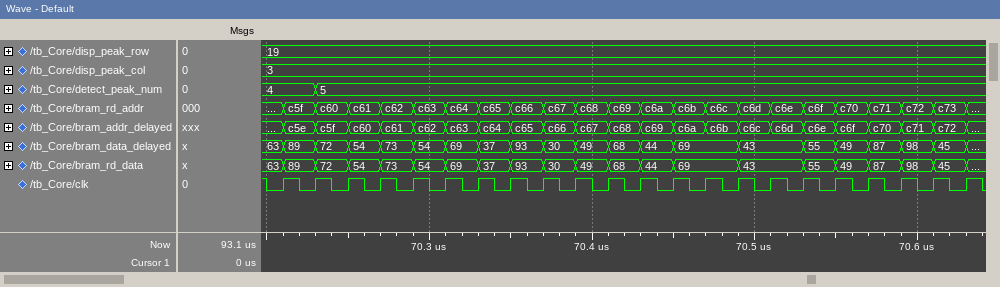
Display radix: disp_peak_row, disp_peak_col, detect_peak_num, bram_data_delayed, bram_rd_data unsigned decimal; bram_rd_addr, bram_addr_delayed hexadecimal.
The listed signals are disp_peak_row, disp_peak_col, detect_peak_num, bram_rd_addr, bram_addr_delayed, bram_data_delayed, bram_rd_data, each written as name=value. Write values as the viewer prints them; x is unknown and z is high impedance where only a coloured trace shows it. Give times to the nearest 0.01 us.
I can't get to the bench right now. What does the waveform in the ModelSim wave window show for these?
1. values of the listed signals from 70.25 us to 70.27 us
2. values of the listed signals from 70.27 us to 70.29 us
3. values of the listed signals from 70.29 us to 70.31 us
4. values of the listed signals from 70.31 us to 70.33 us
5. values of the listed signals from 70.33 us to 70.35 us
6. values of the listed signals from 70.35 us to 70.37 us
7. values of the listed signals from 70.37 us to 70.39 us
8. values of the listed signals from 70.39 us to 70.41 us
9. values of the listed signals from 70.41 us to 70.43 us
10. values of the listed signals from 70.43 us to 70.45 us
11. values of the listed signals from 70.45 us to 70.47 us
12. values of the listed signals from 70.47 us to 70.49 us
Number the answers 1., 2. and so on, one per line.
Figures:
1. disp_peak_row=19, disp_peak_col=3, detect_peak_num=5, bram_rd_addr=c61, bram_addr_delayed=c60, bram_data_delayed=54, bram_rd_data=54
2. disp_peak_row=19, disp_peak_col=3, detect_peak_num=5, bram_rd_addr=c62, bram_addr_delayed=c61, bram_data_delayed=73, bram_rd_data=73
3. disp_peak_row=19, disp_peak_col=3, detect_peak_num=5, bram_rd_addr=c63, bram_addr_delayed=c62, bram_data_delayed=54, bram_rd_data=54
4. disp_peak_row=19, disp_peak_col=3, detect_peak_num=5, bram_rd_addr=c64, bram_addr_delayed=c63, bram_data_delayed=69, bram_rd_data=69
5. disp_peak_row=19, disp_peak_col=3, detect_peak_num=5, bram_rd_addr=c65, bram_addr_delayed=c64, bram_data_delayed=37, bram_rd_data=37
6. disp_peak_row=19, disp_peak_col=3, detect_peak_num=5, bram_rd_addr=c66, bram_addr_delayed=c65, bram_data_delayed=93, bram_rd_data=93
7. disp_peak_row=19, disp_peak_col=3, detect_peak_num=5, bram_rd_addr=c67, bram_addr_delayed=c66, bram_data_delayed=30, bram_rd_data=30
8. disp_peak_row=19, disp_peak_col=3, detect_peak_num=5, bram_rd_addr=c68, bram_addr_delayed=c67, bram_data_delayed=49, bram_rd_data=49
9. disp_peak_row=19, disp_peak_col=3, detect_peak_num=5, bram_rd_addr=c69, bram_addr_delayed=c68, bram_data_delayed=68, bram_rd_data=68
10. disp_peak_row=19, disp_peak_col=3, detect_peak_num=5, bram_rd_addr=c6a, bram_addr_delayed=c69, bram_data_delayed=44, bram_rd_data=44
11. disp_peak_row=19, disp_peak_col=3, detect_peak_num=5, bram_rd_addr=c6b, bram_addr_delayed=c6a, bram_data_delayed=69, bram_rd_data=69
12. disp_peak_row=19, disp_peak_col=3, detect_peak_num=5, bram_rd_addr=c6c, bram_addr_delayed=c6b, bram_data_delayed=69, bram_rd_data=69
